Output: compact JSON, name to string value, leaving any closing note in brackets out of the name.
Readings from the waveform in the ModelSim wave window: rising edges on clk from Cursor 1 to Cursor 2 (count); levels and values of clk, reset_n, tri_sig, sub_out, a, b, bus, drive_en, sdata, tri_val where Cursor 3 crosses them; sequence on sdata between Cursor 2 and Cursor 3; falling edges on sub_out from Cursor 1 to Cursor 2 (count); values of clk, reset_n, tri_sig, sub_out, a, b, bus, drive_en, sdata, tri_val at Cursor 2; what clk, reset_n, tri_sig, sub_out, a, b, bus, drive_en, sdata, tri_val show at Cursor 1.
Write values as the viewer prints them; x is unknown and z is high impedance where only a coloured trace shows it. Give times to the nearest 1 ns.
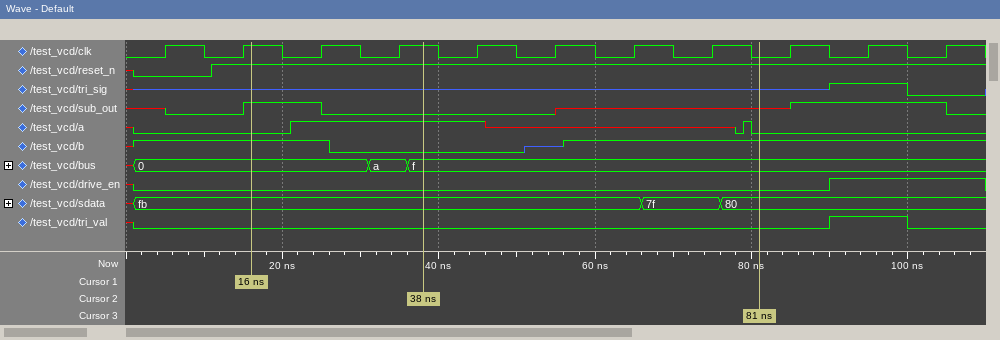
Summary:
{"rising edges on clk from Cursor 1 to Cursor 2": "2", "levels and values of clk, reset_n, tri_sig, sub_out, a, b, bus, drive_en, sdata, tri_val where Cursor 3 crosses them": "clk=0, reset_n=1, tri_sig=z, sub_out=x, a=0, b=1, bus=f, drive_en=0, sdata=80, tri_val=0", "sequence on sdata between Cursor 2 and Cursor 3": "fb, 7f, 80", "falling edges on sub_out from Cursor 1 to Cursor 2": "1", "values of clk, reset_n, tri_sig, sub_out, a, b, bus, drive_en, sdata, tri_val at Cursor 2": "clk=1, reset_n=1, tri_sig=z, sub_out=0, a=1, b=0, bus=f, drive_en=0, sdata=fb, tri_val=0", "what clk, reset_n, tri_sig, sub_out, a, b, bus, drive_en, sdata, tri_val show at Cursor 1": "clk=1, reset_n=1, tri_sig=z, sub_out=1, a=0, b=1, bus=0, drive_en=0, sdata=fb, tri_val=0"}
